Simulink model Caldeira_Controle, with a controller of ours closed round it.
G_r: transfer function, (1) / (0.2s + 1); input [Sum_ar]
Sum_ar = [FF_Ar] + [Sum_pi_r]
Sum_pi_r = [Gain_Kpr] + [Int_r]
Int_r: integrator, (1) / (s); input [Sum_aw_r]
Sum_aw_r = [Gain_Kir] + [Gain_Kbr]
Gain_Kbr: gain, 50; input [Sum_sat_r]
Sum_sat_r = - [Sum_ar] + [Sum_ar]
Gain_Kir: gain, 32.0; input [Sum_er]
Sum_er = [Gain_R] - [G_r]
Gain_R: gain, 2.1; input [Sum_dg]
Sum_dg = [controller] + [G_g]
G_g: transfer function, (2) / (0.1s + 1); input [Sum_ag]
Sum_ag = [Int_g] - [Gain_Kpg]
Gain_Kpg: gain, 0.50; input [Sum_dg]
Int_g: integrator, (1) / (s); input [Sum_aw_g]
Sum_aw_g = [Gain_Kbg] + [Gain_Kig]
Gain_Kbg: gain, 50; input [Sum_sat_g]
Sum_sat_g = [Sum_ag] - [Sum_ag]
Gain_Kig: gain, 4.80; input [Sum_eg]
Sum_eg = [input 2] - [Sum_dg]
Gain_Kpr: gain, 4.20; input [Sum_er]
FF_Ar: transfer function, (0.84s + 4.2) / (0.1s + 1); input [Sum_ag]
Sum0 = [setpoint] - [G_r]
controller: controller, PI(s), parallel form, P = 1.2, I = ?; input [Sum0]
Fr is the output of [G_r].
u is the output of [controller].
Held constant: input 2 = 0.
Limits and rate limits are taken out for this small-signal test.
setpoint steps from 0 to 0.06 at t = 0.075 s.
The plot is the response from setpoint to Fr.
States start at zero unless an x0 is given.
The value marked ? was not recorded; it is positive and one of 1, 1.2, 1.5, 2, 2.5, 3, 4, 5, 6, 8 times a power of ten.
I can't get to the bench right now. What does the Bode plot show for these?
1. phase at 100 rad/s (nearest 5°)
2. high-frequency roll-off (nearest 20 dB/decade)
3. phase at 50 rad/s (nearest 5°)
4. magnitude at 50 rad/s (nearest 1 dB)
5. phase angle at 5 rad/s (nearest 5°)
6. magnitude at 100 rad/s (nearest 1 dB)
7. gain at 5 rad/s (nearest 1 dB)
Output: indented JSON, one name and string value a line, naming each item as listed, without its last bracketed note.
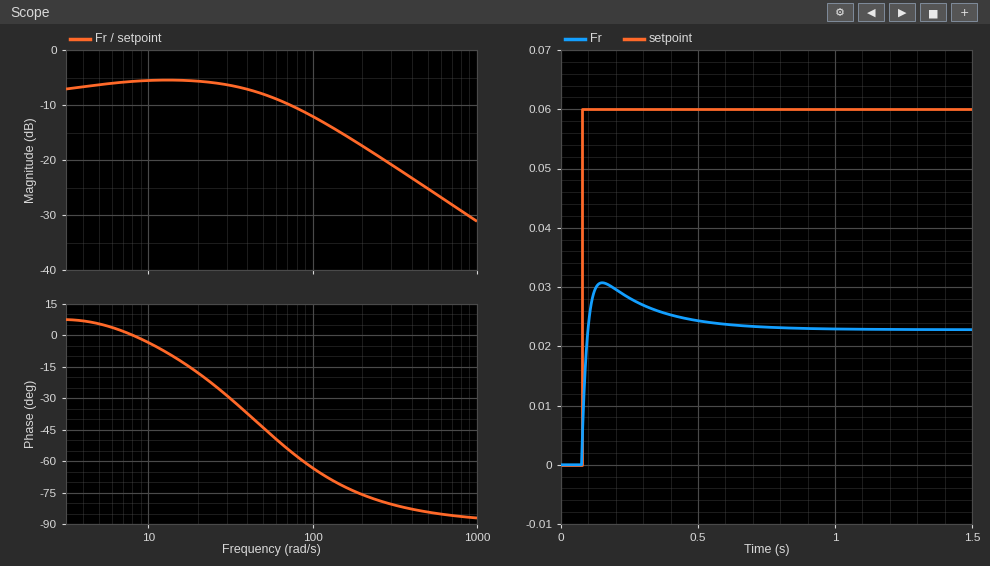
{
  "phase at 100 rad/s": "-65°",
  "high-frequency roll-off": "-20 dB/decade",
  "phase at 50 rad/s": "-45°",
  "magnitude at 50 rad/s": "-8 dB",
  "phase angle at 5 rad/s": "5°",
  "magnitude at 100 rad/s": "-12 dB",
  "gain at 5 rad/s": "-6 dB"
}
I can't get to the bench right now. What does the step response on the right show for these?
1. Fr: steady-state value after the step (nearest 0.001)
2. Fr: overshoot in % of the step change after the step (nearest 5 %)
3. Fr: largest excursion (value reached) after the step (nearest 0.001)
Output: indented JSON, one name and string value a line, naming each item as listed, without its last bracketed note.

{
  "Fr: steady-state value after the step": "0.023",
  "Fr: overshoot in % of the step change after the step": "35 %",
  "Fr: largest excursion (value reached) after the step": "0.031"
}
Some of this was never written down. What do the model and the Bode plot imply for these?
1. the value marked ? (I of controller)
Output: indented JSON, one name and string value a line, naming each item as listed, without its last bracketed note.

{
  "the value marked ?": "4"
}
